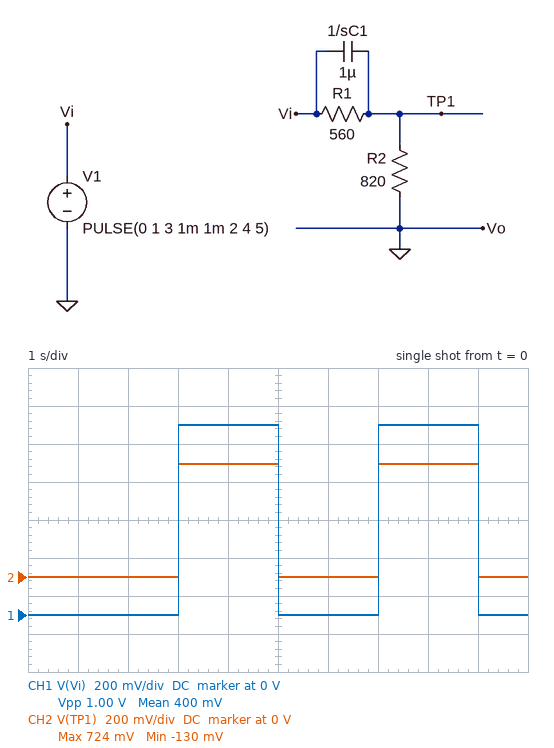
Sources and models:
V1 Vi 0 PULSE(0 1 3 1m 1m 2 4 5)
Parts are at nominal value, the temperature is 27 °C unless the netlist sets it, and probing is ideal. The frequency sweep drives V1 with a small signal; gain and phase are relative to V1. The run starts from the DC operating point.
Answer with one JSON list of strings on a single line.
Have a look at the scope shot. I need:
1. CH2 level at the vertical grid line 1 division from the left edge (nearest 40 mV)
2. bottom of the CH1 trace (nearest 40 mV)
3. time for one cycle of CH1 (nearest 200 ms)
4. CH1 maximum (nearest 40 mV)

["0 V", "0 V", "4.0 s", "1.00 V"]
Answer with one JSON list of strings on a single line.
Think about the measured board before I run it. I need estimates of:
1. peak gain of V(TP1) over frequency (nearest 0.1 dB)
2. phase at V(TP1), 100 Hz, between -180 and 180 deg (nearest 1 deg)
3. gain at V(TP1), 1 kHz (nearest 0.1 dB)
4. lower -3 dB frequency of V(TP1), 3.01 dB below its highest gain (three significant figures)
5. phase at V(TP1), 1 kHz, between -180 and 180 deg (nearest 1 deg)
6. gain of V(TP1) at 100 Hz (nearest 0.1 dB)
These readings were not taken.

["0 dB", "8 deg", "-0.6 dB", "259 Hz", "10 deg", "-4.2 dB"]
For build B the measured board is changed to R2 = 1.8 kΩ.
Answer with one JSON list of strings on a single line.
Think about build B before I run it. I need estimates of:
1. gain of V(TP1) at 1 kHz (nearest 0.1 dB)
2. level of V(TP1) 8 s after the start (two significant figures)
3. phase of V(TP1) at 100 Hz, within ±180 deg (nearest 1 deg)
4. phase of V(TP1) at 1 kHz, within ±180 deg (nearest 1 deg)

["-0.2 dB", "760 mV", "4 deg", "5 deg"]
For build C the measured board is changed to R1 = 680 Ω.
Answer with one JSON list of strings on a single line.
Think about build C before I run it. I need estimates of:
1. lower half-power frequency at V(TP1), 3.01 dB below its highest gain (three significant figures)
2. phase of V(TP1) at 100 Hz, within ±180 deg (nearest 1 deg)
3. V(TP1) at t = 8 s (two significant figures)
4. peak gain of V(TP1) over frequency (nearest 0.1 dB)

["272 Hz", "10 deg", "550 mV", "0 dB"]
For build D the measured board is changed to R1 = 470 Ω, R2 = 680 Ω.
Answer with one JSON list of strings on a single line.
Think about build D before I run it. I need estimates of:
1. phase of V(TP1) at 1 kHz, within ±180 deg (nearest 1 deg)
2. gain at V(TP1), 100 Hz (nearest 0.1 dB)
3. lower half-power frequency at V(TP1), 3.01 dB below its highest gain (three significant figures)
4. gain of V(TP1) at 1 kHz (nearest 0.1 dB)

["11 deg", "-4.3 dB", "314 Hz", "-0.8 dB"]
